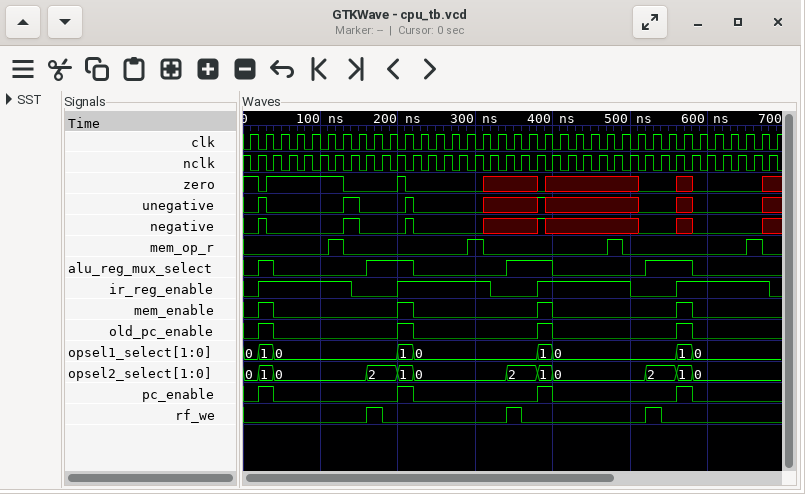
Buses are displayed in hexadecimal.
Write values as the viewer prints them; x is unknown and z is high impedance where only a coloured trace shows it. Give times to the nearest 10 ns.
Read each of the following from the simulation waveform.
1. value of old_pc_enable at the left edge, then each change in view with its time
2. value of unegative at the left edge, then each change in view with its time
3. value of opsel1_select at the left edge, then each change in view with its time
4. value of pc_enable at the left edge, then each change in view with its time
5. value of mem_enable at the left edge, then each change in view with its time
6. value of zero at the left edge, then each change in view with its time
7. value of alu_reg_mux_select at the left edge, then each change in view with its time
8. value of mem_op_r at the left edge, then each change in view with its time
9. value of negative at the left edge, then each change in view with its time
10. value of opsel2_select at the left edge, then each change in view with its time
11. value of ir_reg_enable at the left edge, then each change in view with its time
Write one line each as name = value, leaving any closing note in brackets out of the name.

value of old_pc_enable at the left edge, then each change in view with its time = 0, 1 at 20 ns, 0 at 40 ns, 1 at 200 ns, 0 at 220 ns, 1 at 380 ns, 0 at 400 ns, 1 at 560 ns, 0 at 580 ns
value of unegative at the left edge, then each change in view with its time = 0, 1 at 20 ns, 0 at 30 ns, 1 at 130 ns, 0 at 150 ns, 1 at 210 ns, 0 at 220 ns, x at 310 ns, 1 at 380 ns, x at 390 ns, 0 at 510 ns, x at 560 ns, 0 at 580 ns, x at 670 ns
value of opsel1_select at the left edge, then each change in view with its time = 0, 1 at 20 ns, 0 at 40 ns, 1 at 200 ns, 0 at 220 ns, 1 at 380 ns, 0 at 400 ns, 1 at 560 ns, 0 at 580 ns
value of pc_enable at the left edge, then each change in view with its time = 0, 1 at 20 ns, 0 at 40 ns, 1 at 200 ns, 0 at 220 ns, 1 at 380 ns, 0 at 400 ns, 1 at 560 ns, 0 at 580 ns
value of mem_enable at the left edge, then each change in view with its time = 0, 1 at 20 ns, 0 at 40 ns, 1 at 200 ns, 0 at 220 ns, 1 at 380 ns, 0 at 400 ns, 1 at 560 ns, 0 at 580 ns
value of zero at the left edge, then each change in view with its time = 1, 0 at 20 ns, 1 at 30 ns, 0 at 130 ns, 1 at 200 ns, 0 at 210 ns, x at 310 ns, 0 at 380 ns, x at 390 ns, 0 at 510 ns, x at 560 ns, 0 at 580 ns, x at 670 ns
value of alu_reg_mux_select at the left edge, then each change in view with its time = 0, 1 at 20 ns, 0 at 40 ns, 1 at 160 ns, 0 at 220 ns, 1 at 340 ns, 0 at 400 ns, 1 at 520 ns, 0 at 580 ns
value of mem_op_r at the left edge, then each change in view with its time = 0, 1 at 110 ns, 0 at 130 ns, 1 at 290 ns, 0 at 310 ns, 1 at 470 ns, 0 at 490 ns, 1 at 650 ns, 0 at 670 ns
value of negative at the left edge, then each change in view with its time = 0, 1 at 20 ns, 0 at 30 ns, 1 at 130 ns, 0 at 150 ns, 1 at 210 ns, 0 at 220 ns, x at 310 ns, 1 at 380 ns, x at 390 ns, 0 at 510 ns, x at 560 ns, 0 at 580 ns, x at 670 ns
value of opsel2_select at the left edge, then each change in view with its time = 0, 1 at 20 ns, 0 at 40 ns, 2 at 160 ns, 1 at 200 ns, 0 at 220 ns, 2 at 340 ns, 1 at 380 ns, 0 at 400 ns, 2 at 520 ns, 1 at 560 ns, 0 at 580 ns
value of ir_reg_enable at the left edge, then each change in view with its time = 0, 1 at 20 ns, 0 at 140 ns, 1 at 200 ns, 0 at 320 ns, 1 at 380 ns, 0 at 500 ns, 1 at 560 ns, 0 at 680 ns
